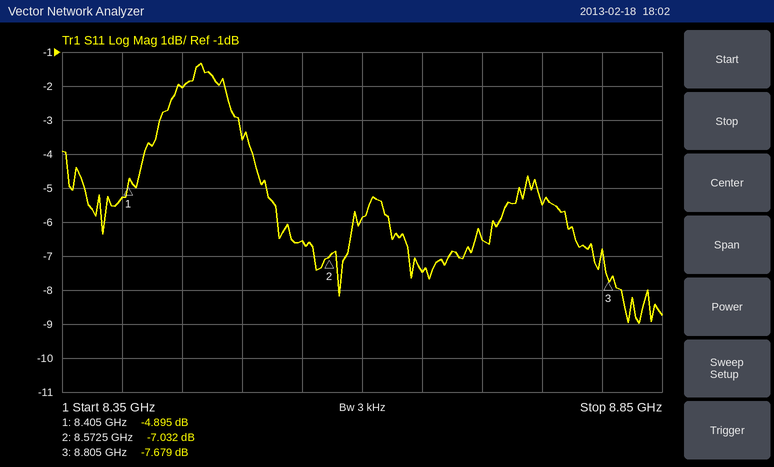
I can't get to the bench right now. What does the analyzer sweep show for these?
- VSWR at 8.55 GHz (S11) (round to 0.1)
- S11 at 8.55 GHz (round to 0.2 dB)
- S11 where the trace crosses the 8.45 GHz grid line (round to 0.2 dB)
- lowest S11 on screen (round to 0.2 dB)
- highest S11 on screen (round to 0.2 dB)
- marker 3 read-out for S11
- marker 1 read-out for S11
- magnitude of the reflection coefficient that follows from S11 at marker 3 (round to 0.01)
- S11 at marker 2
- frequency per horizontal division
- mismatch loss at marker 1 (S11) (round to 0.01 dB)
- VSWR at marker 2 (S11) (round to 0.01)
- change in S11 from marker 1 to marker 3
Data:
2.8
-6.6 dB
-2.0 dB
-9.0 dB
-1.4 dB
-7.679 dB
-4.895 dB
0.41
-7.032 dB
50 MHz
1.70 dB
2.60
-2.784 dB
